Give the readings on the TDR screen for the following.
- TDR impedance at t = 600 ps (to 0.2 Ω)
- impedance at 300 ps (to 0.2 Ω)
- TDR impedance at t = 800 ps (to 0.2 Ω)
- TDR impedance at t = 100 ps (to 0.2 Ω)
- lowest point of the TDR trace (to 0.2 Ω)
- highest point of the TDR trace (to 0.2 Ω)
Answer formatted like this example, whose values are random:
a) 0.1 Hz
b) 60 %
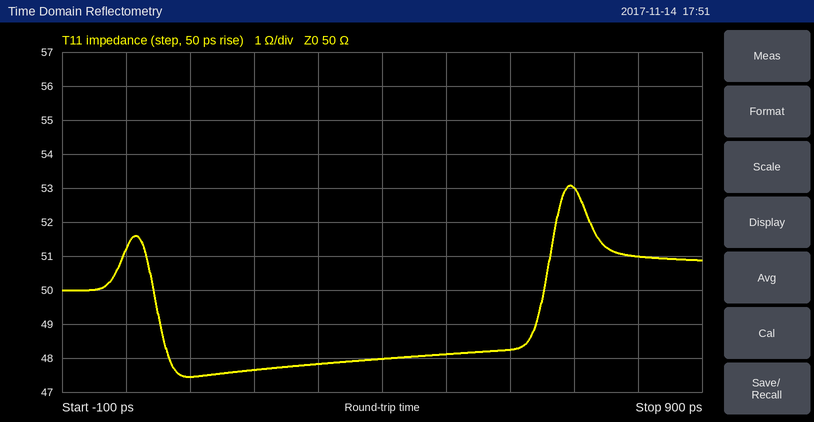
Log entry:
a) 48.2 Ω
b) 47.8 Ω
c) 51.0 Ω
d) 47.4 Ω
e) 47.4 Ω
f) 53.0 Ω
